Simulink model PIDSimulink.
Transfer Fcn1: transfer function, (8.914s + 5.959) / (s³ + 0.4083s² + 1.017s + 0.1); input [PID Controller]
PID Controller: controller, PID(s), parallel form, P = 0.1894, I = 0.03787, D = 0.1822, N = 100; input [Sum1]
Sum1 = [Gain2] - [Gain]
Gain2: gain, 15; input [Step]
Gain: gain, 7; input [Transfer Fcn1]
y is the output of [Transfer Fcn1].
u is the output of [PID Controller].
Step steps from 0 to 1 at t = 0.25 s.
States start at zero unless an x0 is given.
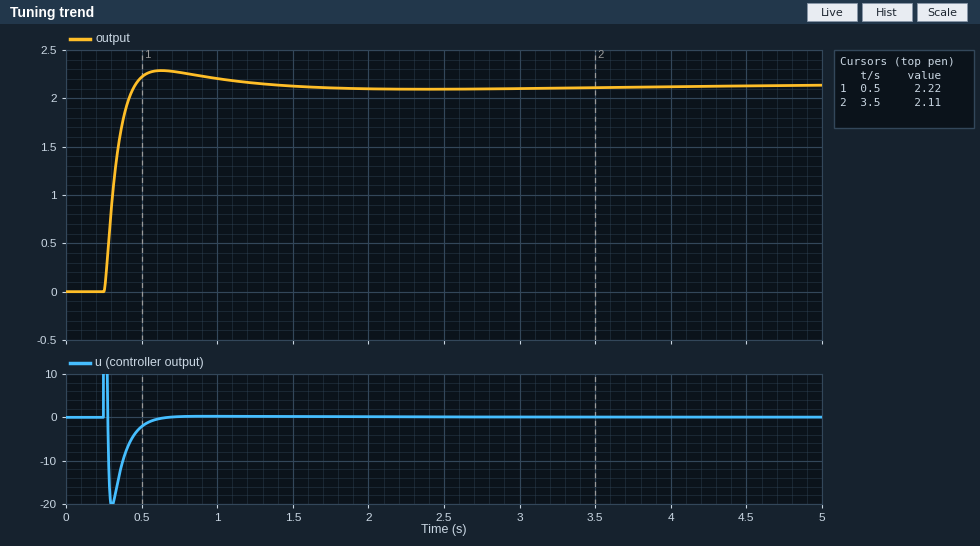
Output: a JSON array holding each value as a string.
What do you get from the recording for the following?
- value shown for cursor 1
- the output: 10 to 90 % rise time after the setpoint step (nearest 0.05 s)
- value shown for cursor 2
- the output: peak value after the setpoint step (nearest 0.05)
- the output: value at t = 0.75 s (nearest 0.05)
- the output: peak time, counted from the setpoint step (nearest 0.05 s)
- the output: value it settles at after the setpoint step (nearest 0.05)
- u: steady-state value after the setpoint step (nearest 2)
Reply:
["2.22", "0.15 s", "2.11", "2.30", "2.25", "0.40 s", "2.15", "0"]
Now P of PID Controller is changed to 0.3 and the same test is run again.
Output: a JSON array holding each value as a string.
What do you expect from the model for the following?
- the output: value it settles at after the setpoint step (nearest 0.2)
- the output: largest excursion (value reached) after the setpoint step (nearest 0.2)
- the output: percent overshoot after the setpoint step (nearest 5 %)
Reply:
["2.2", "2.4", "10 %"]
